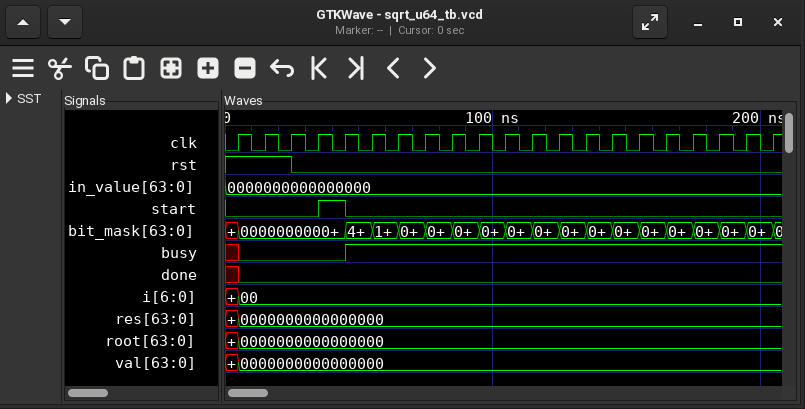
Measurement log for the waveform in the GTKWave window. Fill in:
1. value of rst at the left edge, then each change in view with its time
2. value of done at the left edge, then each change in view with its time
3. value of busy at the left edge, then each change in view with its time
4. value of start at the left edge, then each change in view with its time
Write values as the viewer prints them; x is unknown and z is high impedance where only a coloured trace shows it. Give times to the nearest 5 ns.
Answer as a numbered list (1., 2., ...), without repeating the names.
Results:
1. 1, 0 at 25 ns
2. x, 0 at 5 ns
3. x, 0 at 5 ns, 1 at 45 ns
4. 0, 1 at 35 ns, 0 at 45 ns
